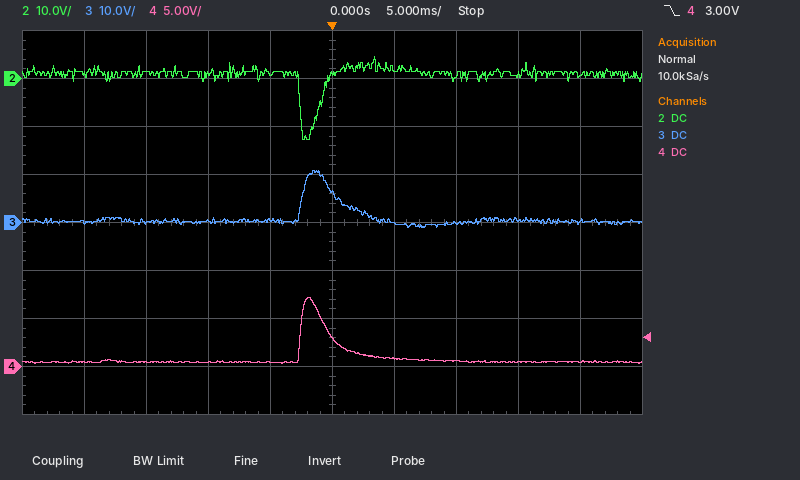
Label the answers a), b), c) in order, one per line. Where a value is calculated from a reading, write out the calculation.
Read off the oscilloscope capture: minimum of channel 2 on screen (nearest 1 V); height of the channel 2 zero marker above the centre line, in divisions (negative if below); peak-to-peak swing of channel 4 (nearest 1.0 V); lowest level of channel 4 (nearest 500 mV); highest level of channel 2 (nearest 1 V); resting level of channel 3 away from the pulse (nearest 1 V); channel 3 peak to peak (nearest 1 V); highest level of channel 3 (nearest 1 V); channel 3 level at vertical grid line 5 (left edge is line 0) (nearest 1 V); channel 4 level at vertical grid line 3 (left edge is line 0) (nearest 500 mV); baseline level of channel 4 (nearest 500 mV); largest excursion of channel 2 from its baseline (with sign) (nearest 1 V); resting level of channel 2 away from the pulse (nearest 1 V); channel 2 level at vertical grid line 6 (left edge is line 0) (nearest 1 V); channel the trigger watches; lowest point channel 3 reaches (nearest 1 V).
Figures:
a) -13 V
b) +3.0 div
c) 7.0 V
d) 500 mV
e) 5 V
f) 0 V
g) 11 V − (-1 V) = 12 V
h) 11 V
i) 6 V
j) 500 mV
k) 500 mV
l) -13 V − (1 V) = -14 V
m) 1 V
n) 2 V
o) channel 4
p) -1 V
